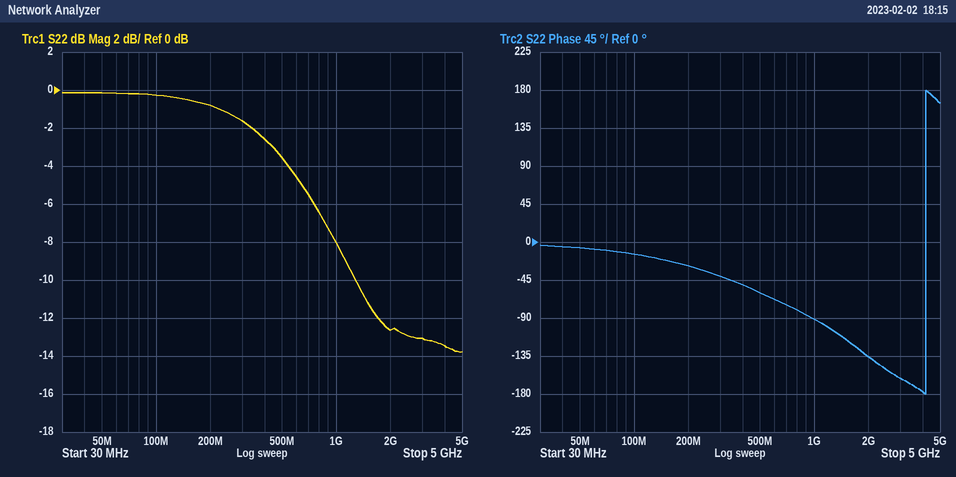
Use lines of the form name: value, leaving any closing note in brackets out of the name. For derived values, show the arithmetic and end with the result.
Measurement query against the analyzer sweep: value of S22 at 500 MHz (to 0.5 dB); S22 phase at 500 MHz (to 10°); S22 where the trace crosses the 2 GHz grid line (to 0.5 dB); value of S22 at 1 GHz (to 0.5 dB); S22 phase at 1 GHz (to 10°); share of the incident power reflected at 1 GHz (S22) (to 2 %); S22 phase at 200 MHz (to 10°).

value of S22 at 500 MHz: -3.5 dB
S22 phase at 500 MHz: -60°
S22 where the trace crosses the 2 GHz grid line: -12.5 dB
value of S22 at 1 GHz: -8.0 dB
S22 phase at 1 GHz: -90°
share of the incident power reflected at 1 GHz (S22): 10^(-8/10) ≈ 16 %
S22 phase at 200 MHz: -30°
